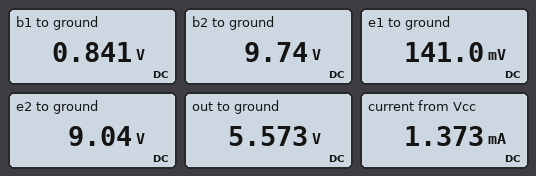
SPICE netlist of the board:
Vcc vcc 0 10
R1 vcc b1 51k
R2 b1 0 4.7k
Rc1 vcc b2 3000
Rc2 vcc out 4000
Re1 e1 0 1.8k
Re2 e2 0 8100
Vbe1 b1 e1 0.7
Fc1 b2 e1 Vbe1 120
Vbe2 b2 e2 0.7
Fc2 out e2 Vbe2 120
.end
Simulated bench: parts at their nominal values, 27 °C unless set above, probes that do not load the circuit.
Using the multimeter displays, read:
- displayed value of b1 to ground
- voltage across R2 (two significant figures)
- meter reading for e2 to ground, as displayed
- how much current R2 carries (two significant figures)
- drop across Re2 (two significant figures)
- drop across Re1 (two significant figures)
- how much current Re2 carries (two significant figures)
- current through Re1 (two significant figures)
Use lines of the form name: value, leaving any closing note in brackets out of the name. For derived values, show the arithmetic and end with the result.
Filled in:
displayed value of b1 to ground: 0.841 V
voltage across R2: 841 mV = 840 mV
meter reading for e2 to ground, as displayed: 9.04 V
how much current R2 carries: (841 mV) / 4.7 kΩ = 180 µA
drop across Re2: 9.04 V = 9.0 V
drop across Re1: 141 mV = 140 mV
how much current Re2 carries: (9.04 V) / 8.1 kΩ = 1.1 mA
current through Re1: (141 mV) / 1.8 kΩ = 78 µA
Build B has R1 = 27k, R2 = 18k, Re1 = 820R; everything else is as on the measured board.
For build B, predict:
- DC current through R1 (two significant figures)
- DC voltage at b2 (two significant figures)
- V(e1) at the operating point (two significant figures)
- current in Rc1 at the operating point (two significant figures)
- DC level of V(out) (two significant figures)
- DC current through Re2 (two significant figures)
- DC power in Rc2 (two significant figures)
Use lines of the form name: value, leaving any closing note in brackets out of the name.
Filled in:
DC current through R1: 230 µA
DC voltage at b2: -790 mV
V(e1) at the operating point: 3.0 V
current in Rc1 at the operating point: 3.6 mA
DC level of V(out): 11 V
DC current through Re2: 180 µA
DC power in Rc2: 130 µW
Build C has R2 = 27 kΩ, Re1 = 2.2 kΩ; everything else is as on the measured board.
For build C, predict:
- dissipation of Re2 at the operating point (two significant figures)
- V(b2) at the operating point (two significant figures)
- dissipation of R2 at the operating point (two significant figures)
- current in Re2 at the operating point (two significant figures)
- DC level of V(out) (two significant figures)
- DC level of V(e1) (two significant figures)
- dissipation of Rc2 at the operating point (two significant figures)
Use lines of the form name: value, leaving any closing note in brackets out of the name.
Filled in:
dissipation of Re2 at the operating point: 4.1 mW
V(b2) at the operating point: 6.5 V
dissipation of R2 at the operating point: 400 µW
current in Re2 at the operating point: 710 µA
DC level of V(out): 7.2 V
DC level of V(e1): 2.6 V
dissipation of Rc2 at the operating point: 2.0 mW
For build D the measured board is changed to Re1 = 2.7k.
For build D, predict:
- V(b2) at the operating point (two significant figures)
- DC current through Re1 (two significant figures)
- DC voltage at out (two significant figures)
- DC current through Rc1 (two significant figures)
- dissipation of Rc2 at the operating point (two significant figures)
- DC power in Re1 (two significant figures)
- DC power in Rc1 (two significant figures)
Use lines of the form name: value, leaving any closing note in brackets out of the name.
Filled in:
V(b2) at the operating point: 9.8 V
DC current through Re1: 53 µA
DC voltage at out: 5.5 V
DC current through Rc1: 61 µA
dissipation of Rc2 at the operating point: 5.0 mW
DC power in Re1: 7.5 µW
DC power in Rc1: 11 µW
